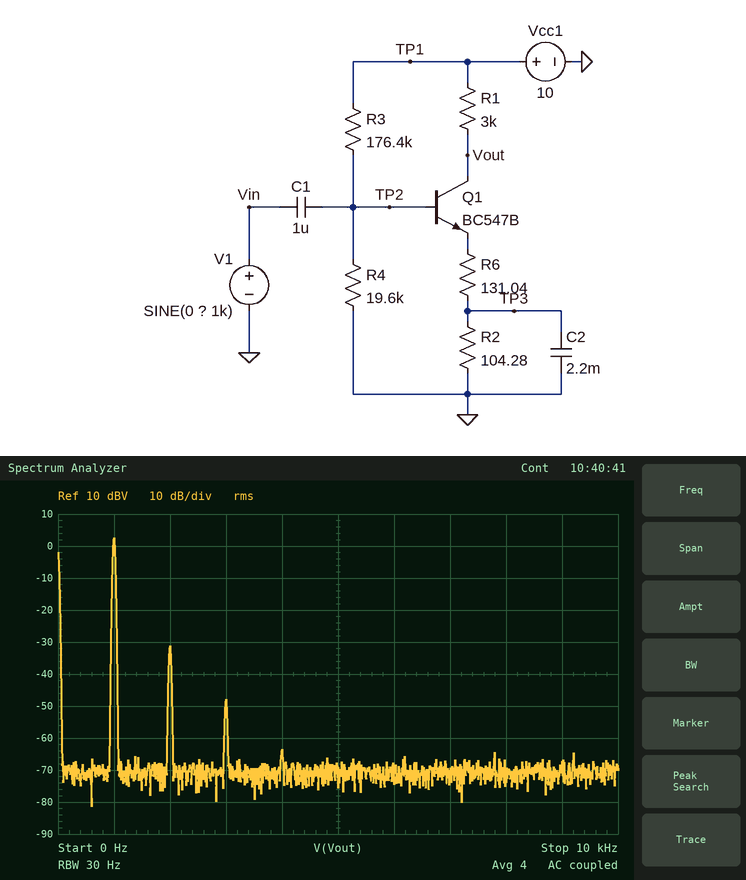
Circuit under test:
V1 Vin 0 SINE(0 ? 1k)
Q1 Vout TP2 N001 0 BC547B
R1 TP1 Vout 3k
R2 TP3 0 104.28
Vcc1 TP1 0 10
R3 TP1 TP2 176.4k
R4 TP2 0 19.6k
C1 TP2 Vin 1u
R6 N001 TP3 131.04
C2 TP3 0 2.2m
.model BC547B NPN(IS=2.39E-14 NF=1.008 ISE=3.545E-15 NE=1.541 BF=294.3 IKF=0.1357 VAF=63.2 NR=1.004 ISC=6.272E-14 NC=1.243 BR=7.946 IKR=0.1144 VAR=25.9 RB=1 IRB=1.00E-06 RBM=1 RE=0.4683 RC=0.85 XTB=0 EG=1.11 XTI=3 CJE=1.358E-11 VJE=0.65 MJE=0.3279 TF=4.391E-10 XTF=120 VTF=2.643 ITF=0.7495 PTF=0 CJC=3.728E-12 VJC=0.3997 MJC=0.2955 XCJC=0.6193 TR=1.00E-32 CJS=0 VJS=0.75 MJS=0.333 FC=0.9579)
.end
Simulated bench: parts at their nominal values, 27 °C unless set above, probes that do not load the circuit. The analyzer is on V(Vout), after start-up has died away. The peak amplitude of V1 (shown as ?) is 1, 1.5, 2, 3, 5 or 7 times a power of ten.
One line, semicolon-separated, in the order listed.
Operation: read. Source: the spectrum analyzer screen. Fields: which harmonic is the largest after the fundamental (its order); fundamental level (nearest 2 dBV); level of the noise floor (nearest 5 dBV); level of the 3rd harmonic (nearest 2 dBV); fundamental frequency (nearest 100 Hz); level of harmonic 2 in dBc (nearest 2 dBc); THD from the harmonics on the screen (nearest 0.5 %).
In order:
2; 2 dBV; -70 dBV; -48 dBV; 1.0 kHz; -34 dBc; 2.0 %
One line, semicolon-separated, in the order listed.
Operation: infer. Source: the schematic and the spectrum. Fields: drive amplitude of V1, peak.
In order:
100 mV
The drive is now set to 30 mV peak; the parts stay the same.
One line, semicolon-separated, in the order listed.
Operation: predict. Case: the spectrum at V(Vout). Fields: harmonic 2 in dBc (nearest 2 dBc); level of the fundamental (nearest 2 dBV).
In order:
-46 dBc; -8 dBV
